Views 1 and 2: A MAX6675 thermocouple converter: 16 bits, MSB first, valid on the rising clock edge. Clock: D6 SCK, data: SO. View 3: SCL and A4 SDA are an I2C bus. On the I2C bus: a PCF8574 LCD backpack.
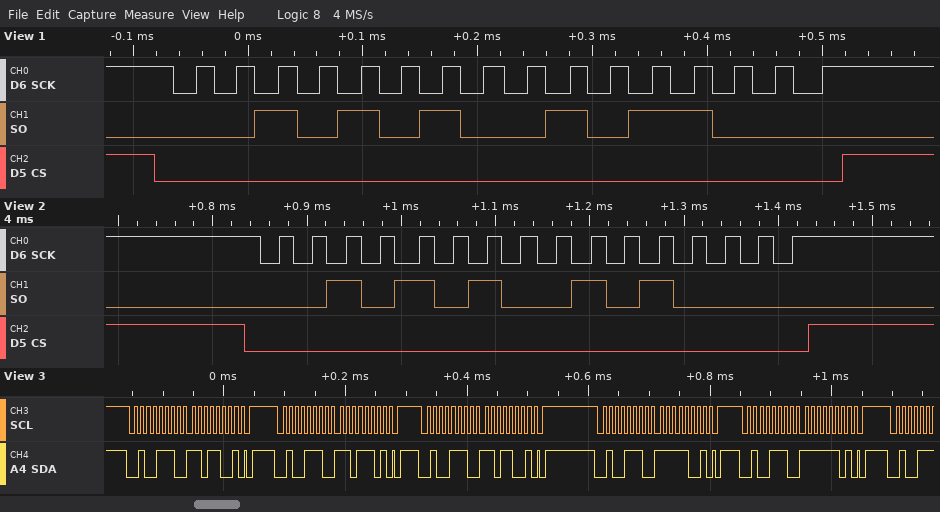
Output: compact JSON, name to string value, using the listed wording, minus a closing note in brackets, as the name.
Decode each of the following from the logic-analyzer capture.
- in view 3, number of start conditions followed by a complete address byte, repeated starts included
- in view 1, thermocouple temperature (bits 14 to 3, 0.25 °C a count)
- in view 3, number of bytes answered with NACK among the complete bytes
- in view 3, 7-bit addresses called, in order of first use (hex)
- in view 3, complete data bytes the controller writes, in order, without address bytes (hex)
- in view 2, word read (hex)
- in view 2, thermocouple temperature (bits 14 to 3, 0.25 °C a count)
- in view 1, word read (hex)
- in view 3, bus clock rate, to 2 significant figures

{"in view 3, number of start conditions followed by a complete address byte, repeated starts included": "5", "in view 1, thermocouple temperature": "338.75 °C", "in view 3, number of bytes answered with NACK among the complete bytes": "0", "in view 3, 7-bit addresses called, in order of first use": "0x27", "in view 3, complete data bytes the controller writes, in order, without address bytes": "D9 DD D9 F9 FD", "in view 2, word read": "0x2A50", "in view 2, thermocouple temperature": "338.50 °C", "in view 1, word read": "0x2A58", "in view 3, bus clock rate, to 2 significant figures": "100 kHz"}
